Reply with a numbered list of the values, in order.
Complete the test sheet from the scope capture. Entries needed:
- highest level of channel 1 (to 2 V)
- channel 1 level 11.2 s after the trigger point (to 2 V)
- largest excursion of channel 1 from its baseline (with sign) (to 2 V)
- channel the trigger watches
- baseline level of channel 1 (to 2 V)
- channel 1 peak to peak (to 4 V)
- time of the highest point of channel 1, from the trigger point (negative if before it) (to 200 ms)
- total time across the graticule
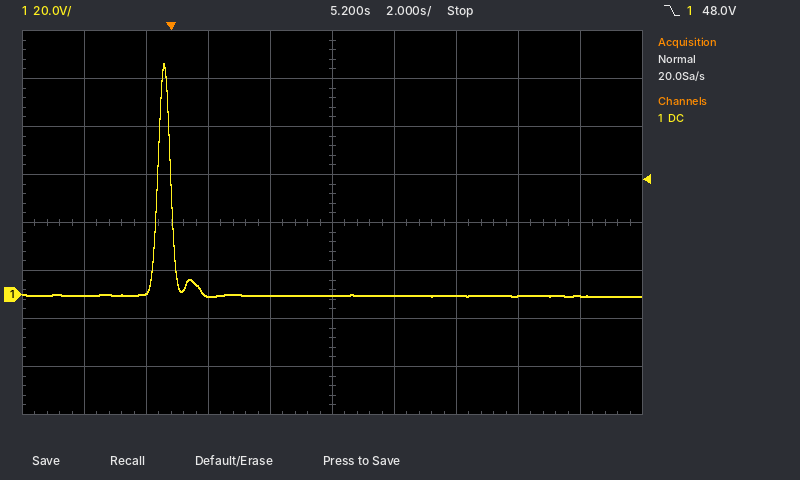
1. 96 V
2. 0 V
3. +96 V
4. channel 1
5. 0 V
6. 96 V
7. -200 ms
8. 20 s
